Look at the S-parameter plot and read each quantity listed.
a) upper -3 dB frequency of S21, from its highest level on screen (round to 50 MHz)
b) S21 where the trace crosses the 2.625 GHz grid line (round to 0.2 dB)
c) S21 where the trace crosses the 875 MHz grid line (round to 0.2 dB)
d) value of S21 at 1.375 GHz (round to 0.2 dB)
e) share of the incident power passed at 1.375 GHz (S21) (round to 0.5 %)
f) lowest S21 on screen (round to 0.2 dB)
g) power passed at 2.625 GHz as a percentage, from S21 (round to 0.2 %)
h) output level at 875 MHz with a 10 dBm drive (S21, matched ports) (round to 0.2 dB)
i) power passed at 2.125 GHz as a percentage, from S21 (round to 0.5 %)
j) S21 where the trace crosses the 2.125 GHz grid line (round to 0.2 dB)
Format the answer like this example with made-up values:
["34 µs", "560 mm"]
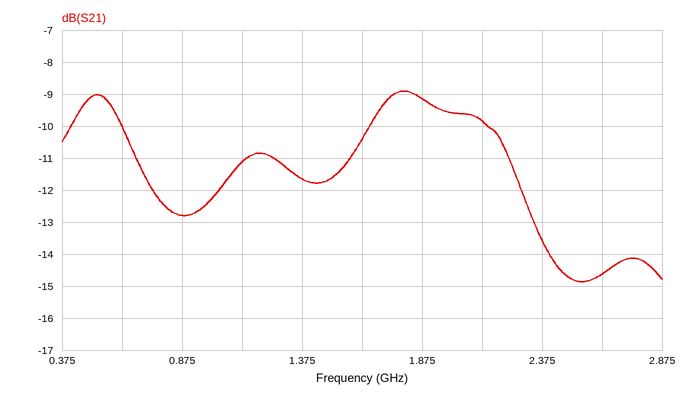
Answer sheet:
["2.30 GHz", "-14.6 dB", "-12.8 dB", "-11.6 dB", "7.0 %", "-14.8 dB", "3.4 %", "-2.8 dBm", "10.5 %", "-9.8 dB"]
